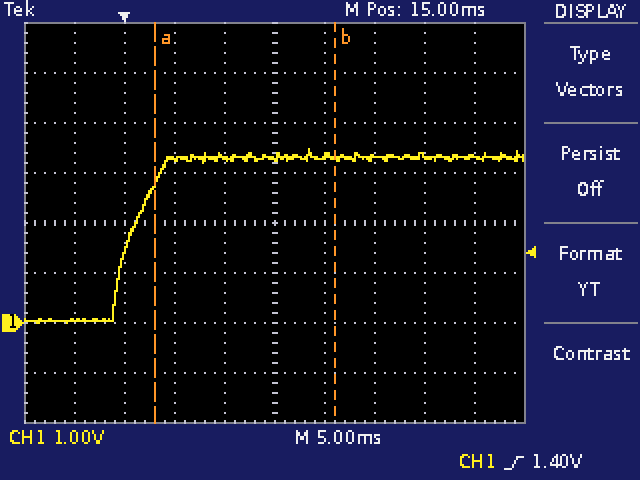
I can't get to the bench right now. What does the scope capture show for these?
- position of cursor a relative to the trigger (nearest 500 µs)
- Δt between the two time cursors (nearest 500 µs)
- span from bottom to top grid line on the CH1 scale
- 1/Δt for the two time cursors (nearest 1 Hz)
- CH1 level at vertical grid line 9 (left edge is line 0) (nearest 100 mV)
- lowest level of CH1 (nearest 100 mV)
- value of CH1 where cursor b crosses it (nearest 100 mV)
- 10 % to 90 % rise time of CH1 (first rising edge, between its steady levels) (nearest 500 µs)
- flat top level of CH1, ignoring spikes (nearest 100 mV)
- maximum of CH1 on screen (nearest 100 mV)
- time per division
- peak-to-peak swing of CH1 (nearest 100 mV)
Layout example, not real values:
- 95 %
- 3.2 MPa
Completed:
- +3.0 ms
- 18.0 ms
- 8 V
- 56 Hz
- 3.3 V
- 0.0 V
- 3.3 V
- 4.5 ms
- 3.3 V
- 3.5 V
- 5 ms
- 3.5 V
